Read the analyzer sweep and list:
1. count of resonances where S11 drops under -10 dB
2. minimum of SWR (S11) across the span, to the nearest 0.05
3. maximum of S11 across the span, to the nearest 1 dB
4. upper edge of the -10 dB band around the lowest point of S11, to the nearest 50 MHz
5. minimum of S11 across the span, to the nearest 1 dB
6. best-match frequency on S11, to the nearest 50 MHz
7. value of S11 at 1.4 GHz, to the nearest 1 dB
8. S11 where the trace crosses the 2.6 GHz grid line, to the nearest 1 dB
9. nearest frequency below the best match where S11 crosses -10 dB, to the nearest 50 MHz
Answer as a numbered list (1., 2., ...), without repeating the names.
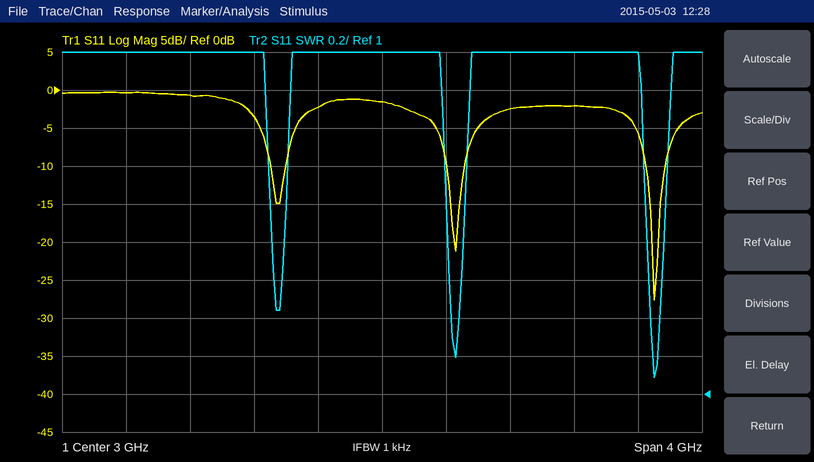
1. 3
2. 1.10
3. 0 dB
4. 4.75 GHz
5. -28 dB
6. 4.70 GHz
7. 0 dB
8. -2 dB
9. 4.65 GHz
